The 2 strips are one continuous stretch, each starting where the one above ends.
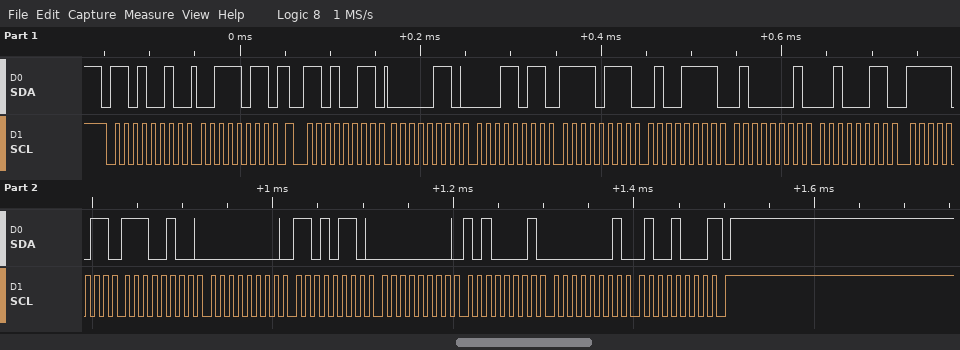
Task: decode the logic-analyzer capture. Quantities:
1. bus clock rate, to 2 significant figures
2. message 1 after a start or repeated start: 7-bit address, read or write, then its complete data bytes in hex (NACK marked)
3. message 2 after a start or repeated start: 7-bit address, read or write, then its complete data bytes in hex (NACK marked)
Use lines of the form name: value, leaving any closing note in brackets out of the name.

bus clock rate, to 2 significant figures: 100 kHz
message 1 after a start or repeated start: 7-bit address, read or write, then its complete data bytes in hex: 0x69 write: 3B
message 2 after a start or repeated start: 7-bit address, read or write, then its complete data bytes in hex: 0x69 read: 06 1B F7 4F 41 23 FB E4 00 D6 00 A1 01 48 NACK
